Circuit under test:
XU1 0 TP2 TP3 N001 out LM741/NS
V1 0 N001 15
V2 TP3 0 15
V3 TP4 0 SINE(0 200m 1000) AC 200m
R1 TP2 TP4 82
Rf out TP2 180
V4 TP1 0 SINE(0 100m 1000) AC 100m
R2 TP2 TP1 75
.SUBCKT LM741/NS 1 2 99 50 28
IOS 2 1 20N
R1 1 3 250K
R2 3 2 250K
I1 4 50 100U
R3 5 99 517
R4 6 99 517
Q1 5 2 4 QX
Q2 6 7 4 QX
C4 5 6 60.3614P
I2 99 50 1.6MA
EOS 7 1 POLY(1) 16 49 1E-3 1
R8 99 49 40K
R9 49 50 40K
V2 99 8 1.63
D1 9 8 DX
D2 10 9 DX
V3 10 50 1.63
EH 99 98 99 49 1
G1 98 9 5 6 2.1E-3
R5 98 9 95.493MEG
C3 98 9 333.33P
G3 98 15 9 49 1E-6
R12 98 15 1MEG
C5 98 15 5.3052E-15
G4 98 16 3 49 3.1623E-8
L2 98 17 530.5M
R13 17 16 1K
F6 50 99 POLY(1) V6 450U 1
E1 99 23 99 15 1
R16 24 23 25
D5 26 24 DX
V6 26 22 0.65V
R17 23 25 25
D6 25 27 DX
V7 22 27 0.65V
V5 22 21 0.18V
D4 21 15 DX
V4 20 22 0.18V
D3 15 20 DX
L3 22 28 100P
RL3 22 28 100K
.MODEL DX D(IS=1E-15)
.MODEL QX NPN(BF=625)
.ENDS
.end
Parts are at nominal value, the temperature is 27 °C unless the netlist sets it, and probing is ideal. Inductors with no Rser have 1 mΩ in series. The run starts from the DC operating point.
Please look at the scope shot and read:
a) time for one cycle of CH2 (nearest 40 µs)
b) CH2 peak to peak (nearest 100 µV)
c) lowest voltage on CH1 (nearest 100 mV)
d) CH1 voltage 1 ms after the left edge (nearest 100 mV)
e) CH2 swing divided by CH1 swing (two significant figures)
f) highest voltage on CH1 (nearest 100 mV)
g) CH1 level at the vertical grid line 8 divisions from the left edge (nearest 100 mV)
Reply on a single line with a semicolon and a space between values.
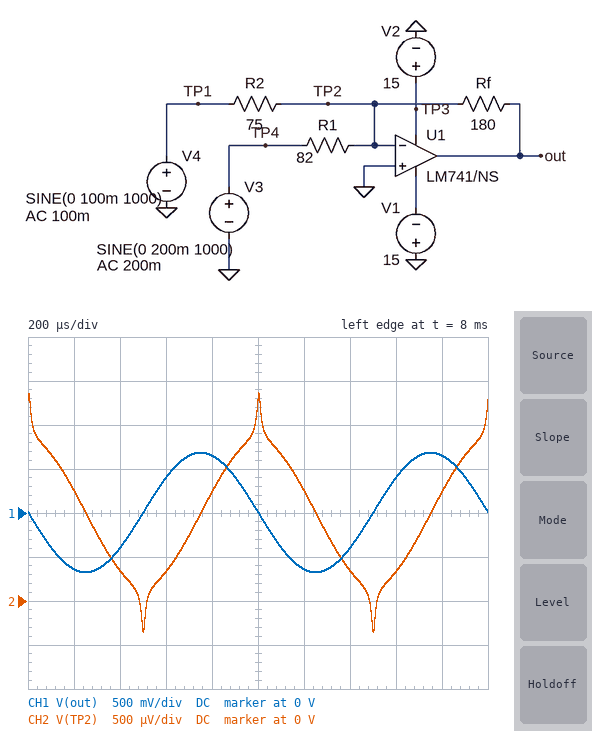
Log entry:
1.00 ms; 2.7 mV; -700 mV; 0 V; 0.0020; 700 mV; 400 mV
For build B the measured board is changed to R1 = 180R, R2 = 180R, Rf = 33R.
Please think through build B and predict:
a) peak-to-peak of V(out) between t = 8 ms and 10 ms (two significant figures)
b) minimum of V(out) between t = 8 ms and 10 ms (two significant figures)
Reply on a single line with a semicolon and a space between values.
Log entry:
110 mV; -54 mV
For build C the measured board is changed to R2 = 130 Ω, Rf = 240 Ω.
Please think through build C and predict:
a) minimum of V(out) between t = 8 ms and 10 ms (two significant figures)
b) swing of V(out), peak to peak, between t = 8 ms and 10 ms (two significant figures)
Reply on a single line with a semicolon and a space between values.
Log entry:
-760 mV; 1.5 V
